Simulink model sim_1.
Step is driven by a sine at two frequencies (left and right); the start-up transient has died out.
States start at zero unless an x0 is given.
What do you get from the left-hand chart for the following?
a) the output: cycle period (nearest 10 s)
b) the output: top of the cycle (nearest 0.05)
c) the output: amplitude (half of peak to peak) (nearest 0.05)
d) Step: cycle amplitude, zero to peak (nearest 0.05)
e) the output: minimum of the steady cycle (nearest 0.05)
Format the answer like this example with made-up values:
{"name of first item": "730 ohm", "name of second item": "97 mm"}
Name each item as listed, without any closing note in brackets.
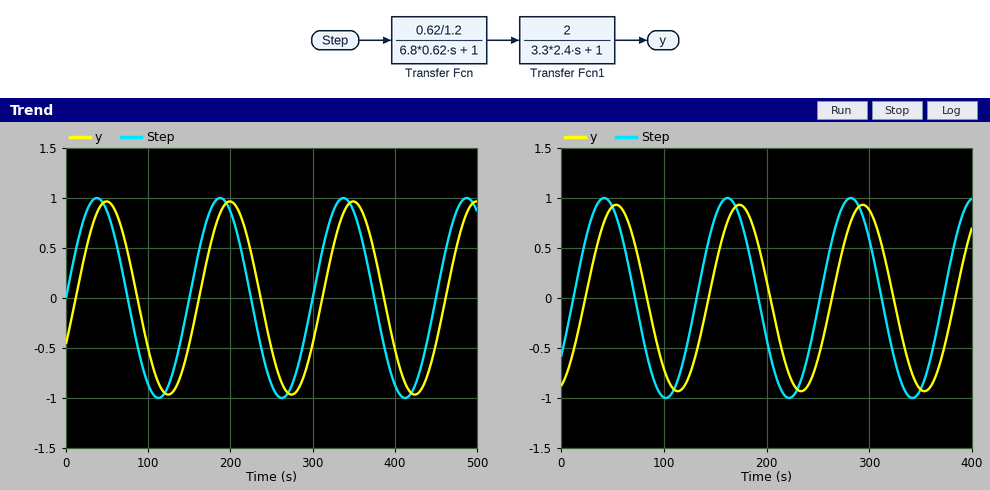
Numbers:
{"the output: cycle period": "150 s", "the output: top of the cycle": "0.95", "the output: amplitude (half of peak to peak)": "0.95", "Step: cycle amplitude, zero to peak": "1.00", "the output: minimum of the steady cycle": "-0.95"}
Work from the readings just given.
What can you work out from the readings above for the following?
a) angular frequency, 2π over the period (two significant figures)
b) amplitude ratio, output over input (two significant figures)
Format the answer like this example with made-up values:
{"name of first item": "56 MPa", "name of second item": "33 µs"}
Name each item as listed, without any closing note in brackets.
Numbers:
{"angular frequency, 2π over the period": "0.042 rad/s", "amplitude ratio, output over input": "0.95"}
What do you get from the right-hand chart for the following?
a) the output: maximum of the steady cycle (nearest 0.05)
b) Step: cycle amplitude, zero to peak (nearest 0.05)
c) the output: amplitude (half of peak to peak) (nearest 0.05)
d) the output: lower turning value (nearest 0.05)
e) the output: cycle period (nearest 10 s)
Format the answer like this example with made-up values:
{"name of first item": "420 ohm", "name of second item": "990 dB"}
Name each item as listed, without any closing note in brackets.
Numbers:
{"the output: maximum of the steady cycle": "0.95", "Step: cycle amplitude, zero to peak": "1.00", "the output: amplitude (half of peak to peak)": "0.95", "the output: lower turning value": "-0.95", "the output: cycle period": "120 s"}
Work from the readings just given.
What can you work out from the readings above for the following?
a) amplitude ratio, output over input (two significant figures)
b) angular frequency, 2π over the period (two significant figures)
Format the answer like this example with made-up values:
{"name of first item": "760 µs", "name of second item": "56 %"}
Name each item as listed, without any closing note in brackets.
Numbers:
{"amplitude ratio, output over input": "0.95", "angular frequency, 2π over the period": "0.052 rad/s"}
